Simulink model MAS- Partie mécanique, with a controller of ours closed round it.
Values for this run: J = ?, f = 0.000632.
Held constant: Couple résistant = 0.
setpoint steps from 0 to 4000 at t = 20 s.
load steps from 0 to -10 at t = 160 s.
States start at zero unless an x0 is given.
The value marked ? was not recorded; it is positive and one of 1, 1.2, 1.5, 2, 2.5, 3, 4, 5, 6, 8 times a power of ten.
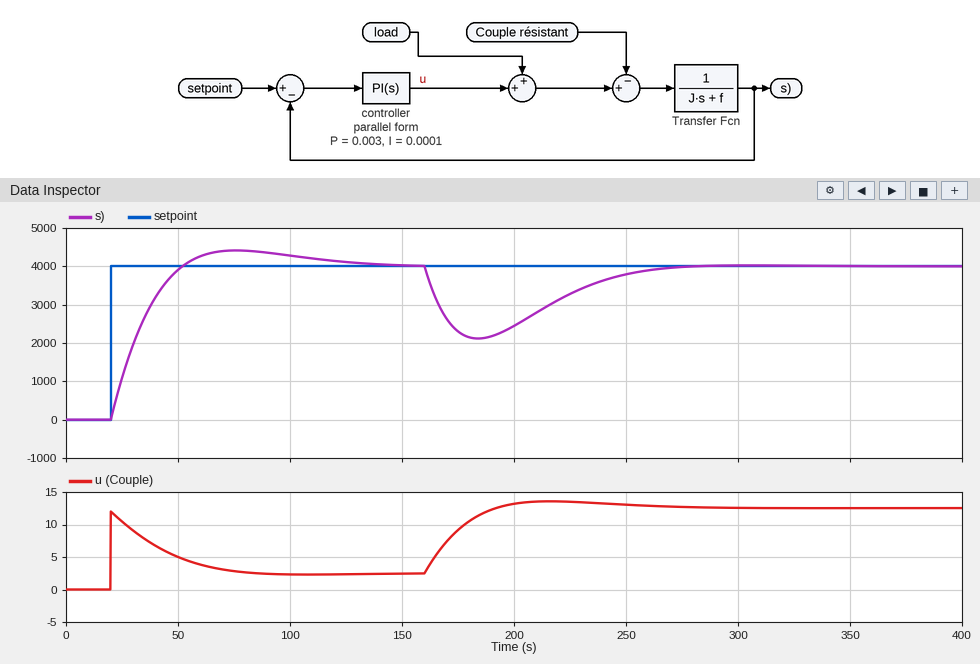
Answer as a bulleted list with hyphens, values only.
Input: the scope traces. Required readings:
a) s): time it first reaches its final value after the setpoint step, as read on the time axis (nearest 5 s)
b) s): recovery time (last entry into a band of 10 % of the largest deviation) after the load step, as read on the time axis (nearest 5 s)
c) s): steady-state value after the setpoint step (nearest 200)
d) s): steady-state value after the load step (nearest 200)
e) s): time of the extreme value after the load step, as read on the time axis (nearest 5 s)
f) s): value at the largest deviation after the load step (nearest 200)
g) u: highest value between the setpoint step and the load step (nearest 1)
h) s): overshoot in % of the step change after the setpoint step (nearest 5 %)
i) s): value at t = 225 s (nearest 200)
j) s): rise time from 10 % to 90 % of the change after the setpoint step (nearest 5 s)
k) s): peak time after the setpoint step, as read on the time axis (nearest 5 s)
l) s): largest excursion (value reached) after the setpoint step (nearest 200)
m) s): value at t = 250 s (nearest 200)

- 50 s
- 250 s
- 4000
- 4000
- 185 s
- 2200
- 12
- 10 %
- 3200
- 25 s
- 75 s
- 4400
- 3800
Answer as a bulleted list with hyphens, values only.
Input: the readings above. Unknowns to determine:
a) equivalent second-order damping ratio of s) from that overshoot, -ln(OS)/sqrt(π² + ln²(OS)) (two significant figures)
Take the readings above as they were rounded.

- 0.59
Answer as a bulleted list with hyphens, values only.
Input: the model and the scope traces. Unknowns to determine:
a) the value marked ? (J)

- 0.05
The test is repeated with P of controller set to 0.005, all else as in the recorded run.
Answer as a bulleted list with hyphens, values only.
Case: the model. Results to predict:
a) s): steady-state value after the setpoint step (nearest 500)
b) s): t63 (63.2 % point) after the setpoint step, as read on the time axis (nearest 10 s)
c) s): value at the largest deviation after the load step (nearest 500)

- 4000
- 30 s
- 2500
